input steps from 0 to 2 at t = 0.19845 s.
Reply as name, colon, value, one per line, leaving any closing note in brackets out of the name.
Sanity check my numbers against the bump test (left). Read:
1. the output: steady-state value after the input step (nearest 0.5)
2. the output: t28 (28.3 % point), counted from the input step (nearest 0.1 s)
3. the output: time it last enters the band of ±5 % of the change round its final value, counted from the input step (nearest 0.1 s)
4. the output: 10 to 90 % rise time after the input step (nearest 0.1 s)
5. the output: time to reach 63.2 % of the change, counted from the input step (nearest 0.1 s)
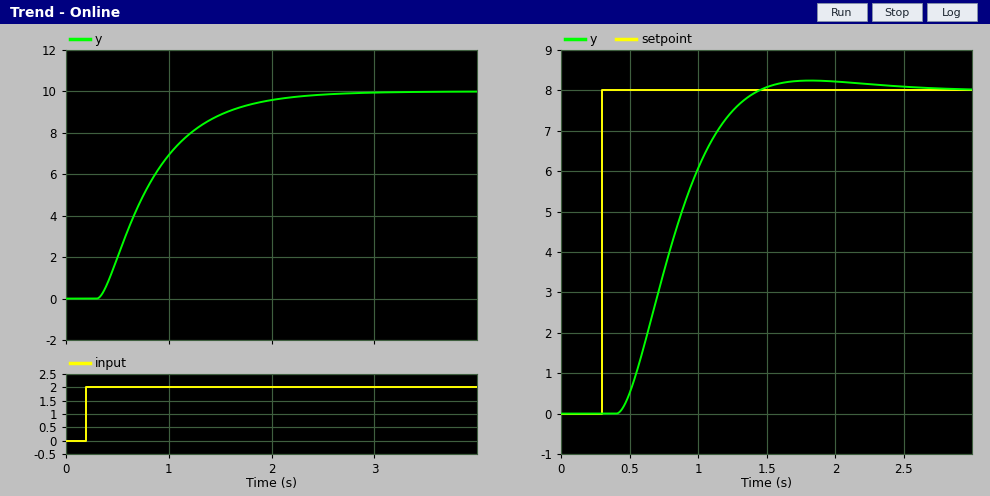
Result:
the output: steady-state value after the input step: 10.0
the output: t28 (28.3 % point), counted from the input step: 0.4 s
the output: time it last enters the band of ±5 % of the change round its final value, counted from the input step: 1.7 s
the output: 10 to 90 % rise time after the input step: 1.1 s
the output: time to reach 63.2 % of the change, counted from the input step: 0.7 s
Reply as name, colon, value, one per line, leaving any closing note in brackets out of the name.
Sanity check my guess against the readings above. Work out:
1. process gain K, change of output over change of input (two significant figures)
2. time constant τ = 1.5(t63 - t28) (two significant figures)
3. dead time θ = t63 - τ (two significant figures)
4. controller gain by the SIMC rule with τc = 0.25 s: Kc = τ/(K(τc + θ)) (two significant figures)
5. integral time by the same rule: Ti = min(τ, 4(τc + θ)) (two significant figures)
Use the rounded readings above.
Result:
process gain K, change of output over change of input: 5.0
time constant τ = 1.5(t63 - t28): 0.45 s
dead time θ = t63 - τ: 0.25 s
controller gain by the SIMC rule with τc = 0.25 s: Kc = τ/(K(τc + θ)): 0.18
integral time by the same rule: Ti = min(τ, 4(τc + θ)): 0.45 s
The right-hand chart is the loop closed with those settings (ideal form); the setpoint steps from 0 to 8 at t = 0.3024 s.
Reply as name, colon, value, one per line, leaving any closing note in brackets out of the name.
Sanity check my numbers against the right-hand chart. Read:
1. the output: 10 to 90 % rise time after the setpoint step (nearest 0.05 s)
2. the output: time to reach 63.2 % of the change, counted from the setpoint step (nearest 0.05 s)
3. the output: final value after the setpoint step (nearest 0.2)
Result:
the output: 10 to 90 % rise time after the setpoint step: 0.65 s
the output: time to reach 63.2 % of the change, counted from the setpoint step: 0.60 s
the output: final value after the setpoint step: 8.0
